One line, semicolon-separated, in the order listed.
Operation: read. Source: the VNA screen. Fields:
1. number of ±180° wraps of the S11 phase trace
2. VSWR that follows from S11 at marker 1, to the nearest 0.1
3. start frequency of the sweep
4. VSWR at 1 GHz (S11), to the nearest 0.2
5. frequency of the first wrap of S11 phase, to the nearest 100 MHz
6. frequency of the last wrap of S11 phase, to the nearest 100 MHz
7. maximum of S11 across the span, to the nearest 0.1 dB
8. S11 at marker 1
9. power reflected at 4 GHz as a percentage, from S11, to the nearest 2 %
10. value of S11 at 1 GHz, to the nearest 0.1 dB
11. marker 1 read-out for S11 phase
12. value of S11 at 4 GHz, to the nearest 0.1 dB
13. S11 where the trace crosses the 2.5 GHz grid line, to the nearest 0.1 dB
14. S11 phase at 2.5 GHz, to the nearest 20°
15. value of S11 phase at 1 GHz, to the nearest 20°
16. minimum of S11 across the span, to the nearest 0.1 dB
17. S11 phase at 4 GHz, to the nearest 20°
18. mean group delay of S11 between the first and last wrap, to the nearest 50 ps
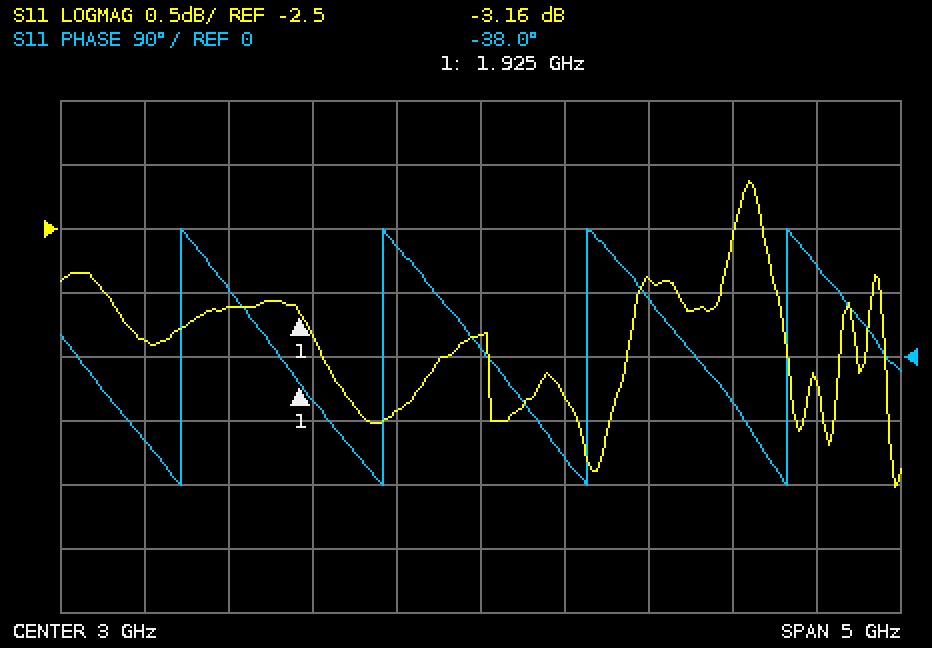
4; 5.6; 500 MHz; 5.2; 1.2 GHz; 4.8 GHz; -2.1 dB; -3.16 dB; 52 %; -3.4 dB; -38.0°; -2.9 dB; -3.9 dB; 160°; -120°; -4.5 dB; 80°; 850 ps
